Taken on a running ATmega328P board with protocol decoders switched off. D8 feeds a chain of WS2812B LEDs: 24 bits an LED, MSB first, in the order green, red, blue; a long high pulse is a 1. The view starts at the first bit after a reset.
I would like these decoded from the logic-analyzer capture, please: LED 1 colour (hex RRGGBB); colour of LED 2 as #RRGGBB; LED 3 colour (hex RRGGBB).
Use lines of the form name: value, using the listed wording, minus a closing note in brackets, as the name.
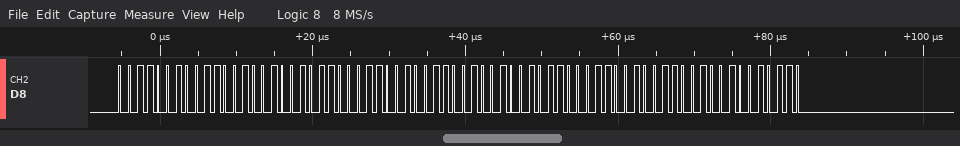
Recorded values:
LED 1 colour: #643296
colour of LED 2 as #RRGGBB: #643296
LED 3 colour: #643296
